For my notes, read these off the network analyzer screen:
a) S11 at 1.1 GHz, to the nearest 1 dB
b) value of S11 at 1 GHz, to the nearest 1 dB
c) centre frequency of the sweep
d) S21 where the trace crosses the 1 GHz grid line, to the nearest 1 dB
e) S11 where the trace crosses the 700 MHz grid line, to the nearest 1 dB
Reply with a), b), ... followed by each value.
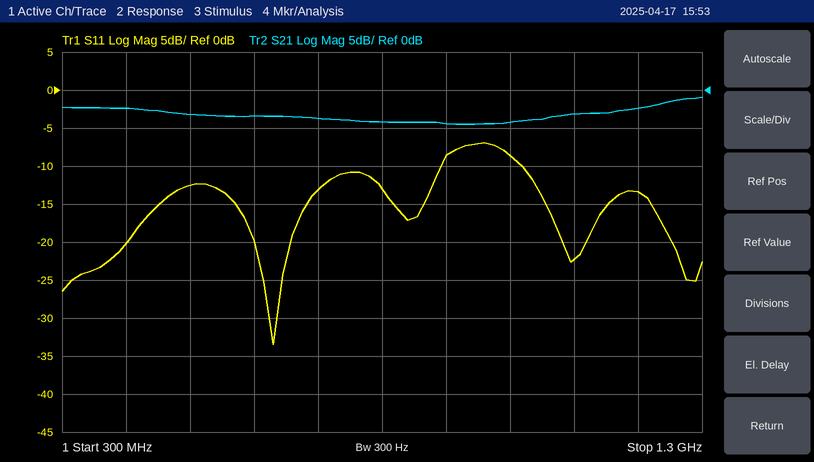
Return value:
a) -22 dB
b) -9 dB
c) 800 MHz
d) -4 dB
e) -13 dB
